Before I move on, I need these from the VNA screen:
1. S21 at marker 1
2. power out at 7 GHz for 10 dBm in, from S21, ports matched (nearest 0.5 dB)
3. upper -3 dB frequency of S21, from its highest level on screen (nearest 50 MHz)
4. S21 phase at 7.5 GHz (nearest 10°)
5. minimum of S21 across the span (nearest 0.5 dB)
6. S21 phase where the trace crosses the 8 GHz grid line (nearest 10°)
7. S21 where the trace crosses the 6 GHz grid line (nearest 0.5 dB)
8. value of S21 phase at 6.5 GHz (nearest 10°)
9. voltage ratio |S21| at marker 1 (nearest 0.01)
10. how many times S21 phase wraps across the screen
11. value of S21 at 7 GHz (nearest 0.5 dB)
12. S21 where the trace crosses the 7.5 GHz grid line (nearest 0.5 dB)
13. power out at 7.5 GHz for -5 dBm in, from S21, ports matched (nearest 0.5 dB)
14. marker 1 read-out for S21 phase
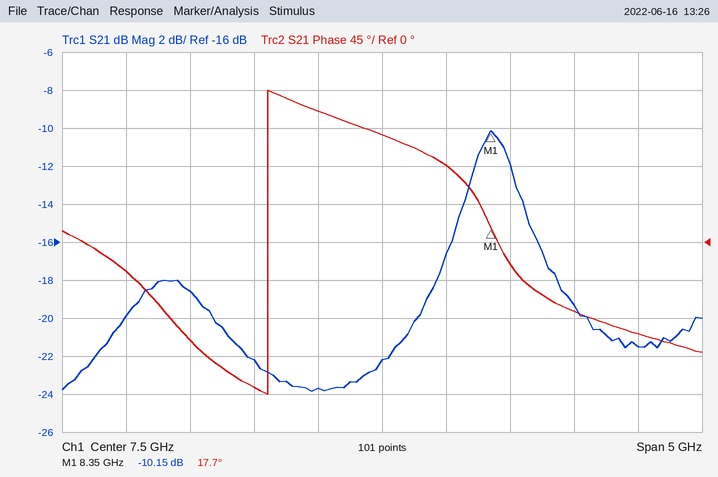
-10.15 dB
-13.5 dBm
8.55 GHz
130°
-24.0 dB
90°
-18.5 dB
-170°
0.31
1
-23.5 dB
-22.0 dB
-27.0 dBm
17.7°
